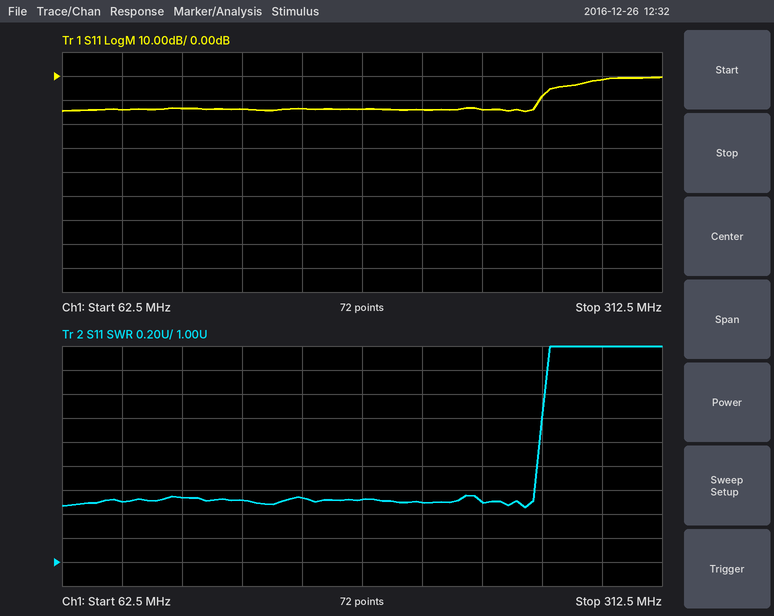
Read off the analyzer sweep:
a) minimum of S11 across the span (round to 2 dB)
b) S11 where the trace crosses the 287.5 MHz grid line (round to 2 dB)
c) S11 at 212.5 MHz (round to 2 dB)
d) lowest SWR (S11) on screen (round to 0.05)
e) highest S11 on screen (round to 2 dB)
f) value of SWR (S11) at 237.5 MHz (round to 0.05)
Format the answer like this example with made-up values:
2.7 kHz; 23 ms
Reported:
-14 dB; -2 dB; -14 dB; 1.45; 0 dB; 1.50
